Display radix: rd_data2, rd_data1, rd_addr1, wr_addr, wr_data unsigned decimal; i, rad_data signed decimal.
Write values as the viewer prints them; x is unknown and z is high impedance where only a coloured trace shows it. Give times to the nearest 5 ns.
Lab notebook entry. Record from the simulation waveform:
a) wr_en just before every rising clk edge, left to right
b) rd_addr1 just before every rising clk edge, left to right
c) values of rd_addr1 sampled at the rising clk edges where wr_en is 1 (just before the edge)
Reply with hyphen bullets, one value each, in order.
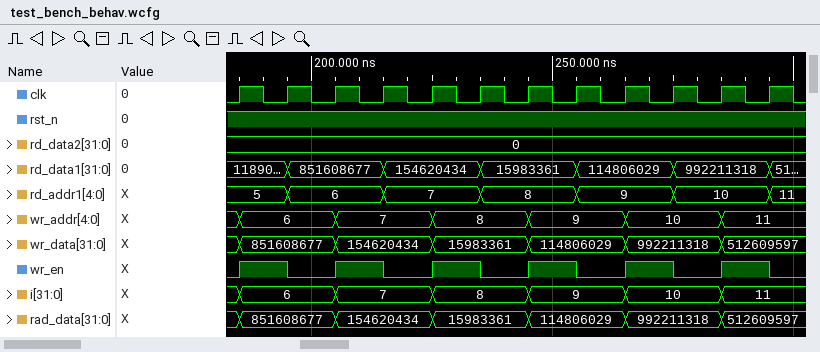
- 0 1 0 1 0 1 0 1 0 1 0 1
- 5, 5, 6, 6, 7, 7, 8, 8, 9, 9, 10, 10
- 5, 6, 7, 8, 9, 10
